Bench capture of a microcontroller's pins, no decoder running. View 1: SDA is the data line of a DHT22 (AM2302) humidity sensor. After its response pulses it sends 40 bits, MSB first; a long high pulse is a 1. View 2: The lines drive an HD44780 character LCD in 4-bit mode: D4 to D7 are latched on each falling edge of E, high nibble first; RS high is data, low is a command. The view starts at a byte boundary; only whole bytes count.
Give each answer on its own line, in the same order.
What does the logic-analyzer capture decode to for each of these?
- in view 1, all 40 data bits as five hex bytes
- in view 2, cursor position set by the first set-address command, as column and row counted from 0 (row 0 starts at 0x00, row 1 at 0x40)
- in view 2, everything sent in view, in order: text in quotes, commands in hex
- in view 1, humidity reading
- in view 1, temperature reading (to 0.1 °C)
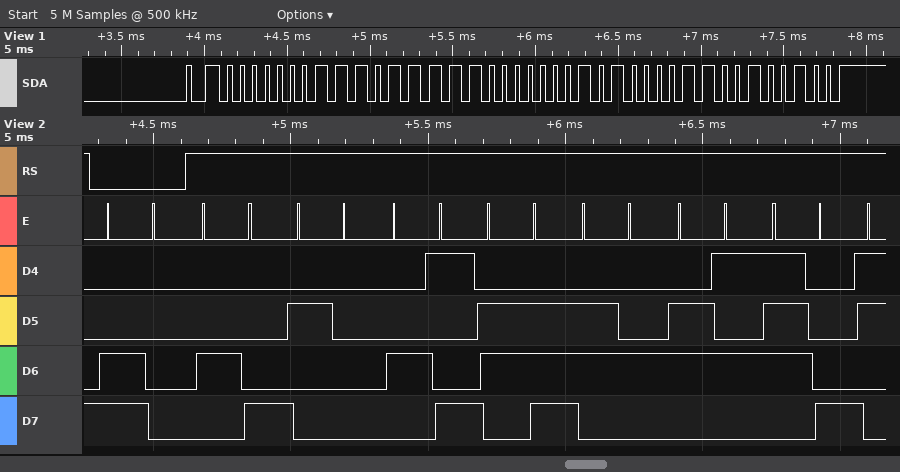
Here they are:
01 DF 01 43 24
column 0, row 1
0xC0 "H Index"
47.9 %
32.3 °C
